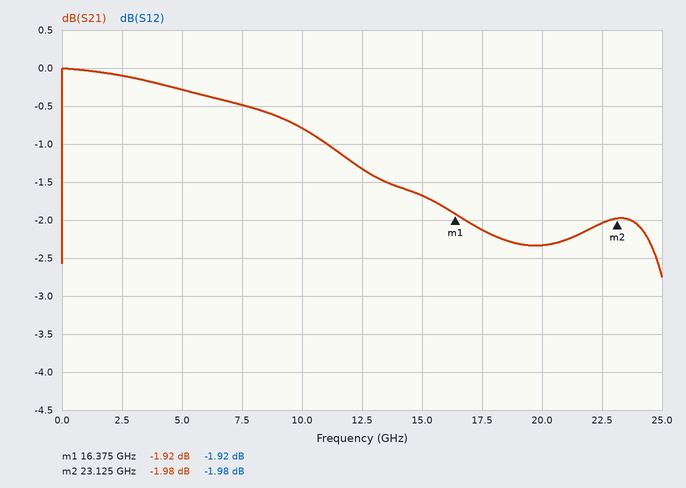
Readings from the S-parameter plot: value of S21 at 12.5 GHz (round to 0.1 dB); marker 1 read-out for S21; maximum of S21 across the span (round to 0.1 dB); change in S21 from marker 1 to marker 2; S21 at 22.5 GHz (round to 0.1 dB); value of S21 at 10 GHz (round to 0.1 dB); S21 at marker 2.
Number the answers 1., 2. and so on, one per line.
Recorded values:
1. -1.3 dB
2. -1.92 dB
3. 0.0 dB
4. -0.06 dB
5. -2.0 dB
6. -0.8 dB
7. -1.98 dB
